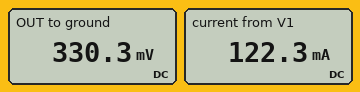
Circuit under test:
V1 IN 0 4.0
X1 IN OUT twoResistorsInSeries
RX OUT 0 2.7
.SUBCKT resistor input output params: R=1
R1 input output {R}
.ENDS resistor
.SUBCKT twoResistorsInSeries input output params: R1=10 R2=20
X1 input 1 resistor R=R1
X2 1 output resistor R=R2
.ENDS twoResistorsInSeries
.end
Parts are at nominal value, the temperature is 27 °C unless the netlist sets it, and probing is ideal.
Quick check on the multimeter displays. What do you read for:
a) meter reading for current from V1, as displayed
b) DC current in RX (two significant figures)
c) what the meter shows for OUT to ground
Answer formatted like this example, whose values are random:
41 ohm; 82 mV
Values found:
122.3 mA; 120 mA; 330.3 mV
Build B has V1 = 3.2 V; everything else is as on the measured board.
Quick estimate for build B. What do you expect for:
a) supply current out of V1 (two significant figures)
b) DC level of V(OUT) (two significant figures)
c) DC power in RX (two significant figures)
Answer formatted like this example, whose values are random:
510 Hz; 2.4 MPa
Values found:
98 mA; 260 mV; 26 mW
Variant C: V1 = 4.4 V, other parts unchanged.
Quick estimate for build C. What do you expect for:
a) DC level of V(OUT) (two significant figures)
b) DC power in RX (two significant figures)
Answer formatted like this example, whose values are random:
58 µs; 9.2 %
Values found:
360 mV; 49 mW
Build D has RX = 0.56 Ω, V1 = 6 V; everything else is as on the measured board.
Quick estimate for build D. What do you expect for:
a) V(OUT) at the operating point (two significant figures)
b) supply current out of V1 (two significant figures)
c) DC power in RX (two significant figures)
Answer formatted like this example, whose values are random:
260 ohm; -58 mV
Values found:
110 mV; 200 mA; 22 mW
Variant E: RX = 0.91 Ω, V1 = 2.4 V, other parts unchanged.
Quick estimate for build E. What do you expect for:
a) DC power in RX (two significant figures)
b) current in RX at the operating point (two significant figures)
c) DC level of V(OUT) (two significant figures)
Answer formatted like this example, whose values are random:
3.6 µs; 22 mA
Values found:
5.5 mW; 78 mA; 71 mV
